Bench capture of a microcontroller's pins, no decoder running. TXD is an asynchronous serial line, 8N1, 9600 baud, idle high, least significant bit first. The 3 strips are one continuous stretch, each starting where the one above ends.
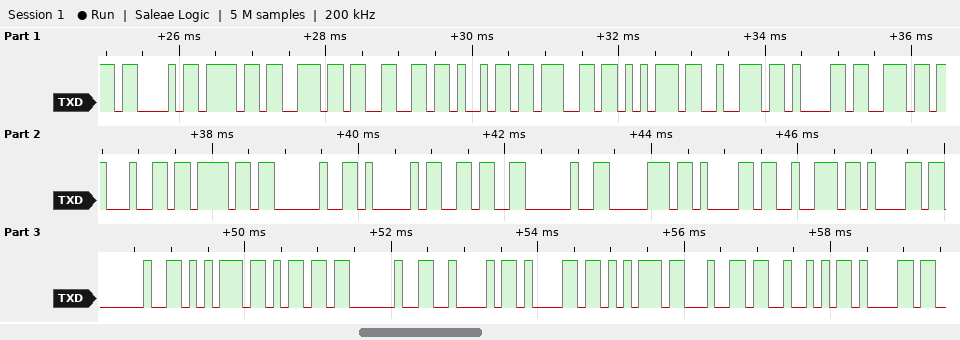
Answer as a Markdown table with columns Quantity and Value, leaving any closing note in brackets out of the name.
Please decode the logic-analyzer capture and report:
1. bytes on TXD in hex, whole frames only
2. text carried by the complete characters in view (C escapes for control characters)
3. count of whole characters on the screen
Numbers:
| Quantity | Value |
|---|---|
| bytes on TXD in hex, whole frames only | 43 6F 6E 66 69 67 75 72 61 6E 64 6F 20 41 36 20 70 61 72 61 20 75 6D 20 42 61 75 64 52 61 |
| text carried by the complete characters in view | "Configurando A6 para um BaudRa" |
| count of whole characters on the screen | 30 |
